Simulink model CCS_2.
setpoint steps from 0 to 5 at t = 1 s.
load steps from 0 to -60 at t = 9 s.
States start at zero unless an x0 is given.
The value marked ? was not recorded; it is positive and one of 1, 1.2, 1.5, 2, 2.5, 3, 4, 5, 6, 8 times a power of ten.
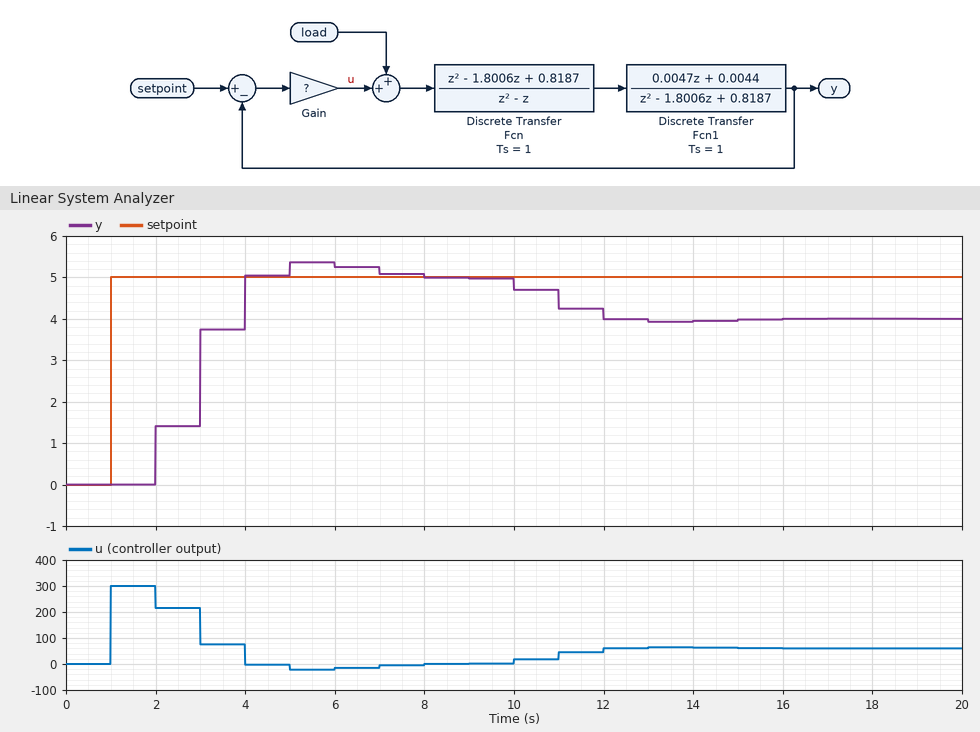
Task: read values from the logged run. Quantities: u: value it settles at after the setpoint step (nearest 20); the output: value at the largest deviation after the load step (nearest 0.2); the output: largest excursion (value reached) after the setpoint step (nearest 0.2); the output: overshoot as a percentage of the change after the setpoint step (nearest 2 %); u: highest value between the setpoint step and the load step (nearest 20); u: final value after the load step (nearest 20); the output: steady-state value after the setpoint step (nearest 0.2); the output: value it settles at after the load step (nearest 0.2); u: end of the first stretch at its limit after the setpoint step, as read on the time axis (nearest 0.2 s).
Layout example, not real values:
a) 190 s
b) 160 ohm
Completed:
a) 0
b) 4.0
c) 5.4
d) 8 %
e) 300
f) 60
g) 5.0
h) 4.0
i) 2.0 s
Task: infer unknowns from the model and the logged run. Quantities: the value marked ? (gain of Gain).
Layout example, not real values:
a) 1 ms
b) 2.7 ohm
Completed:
a) 60
